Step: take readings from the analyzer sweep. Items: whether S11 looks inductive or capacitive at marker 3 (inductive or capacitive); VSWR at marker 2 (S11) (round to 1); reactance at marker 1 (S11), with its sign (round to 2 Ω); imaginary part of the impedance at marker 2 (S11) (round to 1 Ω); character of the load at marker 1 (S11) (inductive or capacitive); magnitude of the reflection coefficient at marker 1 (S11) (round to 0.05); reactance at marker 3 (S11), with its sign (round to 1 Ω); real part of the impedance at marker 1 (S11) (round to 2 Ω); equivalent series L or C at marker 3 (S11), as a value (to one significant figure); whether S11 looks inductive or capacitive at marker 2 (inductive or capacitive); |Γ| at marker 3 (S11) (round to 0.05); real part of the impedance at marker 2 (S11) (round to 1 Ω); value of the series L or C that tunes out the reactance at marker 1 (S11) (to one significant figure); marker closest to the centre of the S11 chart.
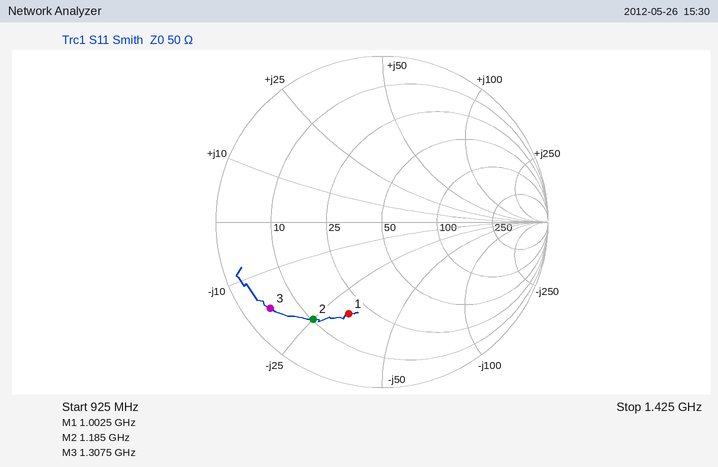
capacitive
6
-32 Ω
-25 Ω
capacitive
0.60
-17 Ω
18 Ω
7 pF
capacitive
0.85
10 Ω
5 nH
marker 1
